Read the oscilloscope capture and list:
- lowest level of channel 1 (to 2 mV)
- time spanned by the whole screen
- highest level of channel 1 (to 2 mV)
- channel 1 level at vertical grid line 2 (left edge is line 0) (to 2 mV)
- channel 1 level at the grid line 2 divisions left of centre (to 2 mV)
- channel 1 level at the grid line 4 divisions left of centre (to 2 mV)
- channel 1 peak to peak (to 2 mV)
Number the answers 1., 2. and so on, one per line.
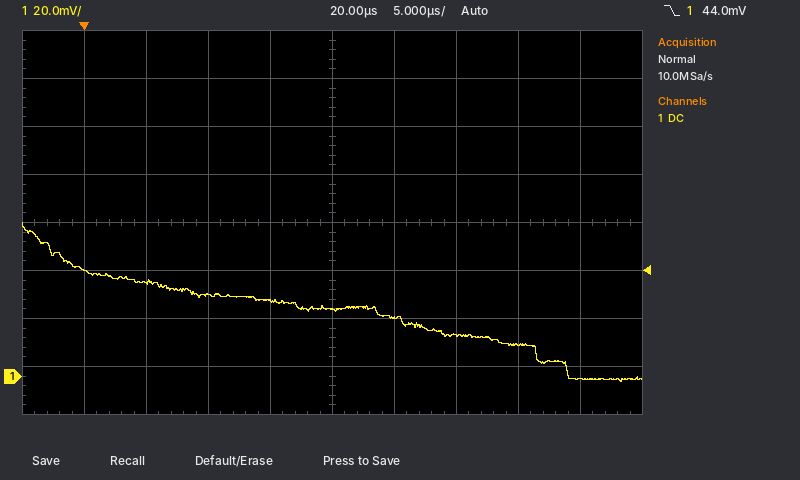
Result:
1. -2 mV
2. 50 µs
3. 64 mV
4. 40 mV
5. 34 mV
6. 44 mV
7. 66 mV
